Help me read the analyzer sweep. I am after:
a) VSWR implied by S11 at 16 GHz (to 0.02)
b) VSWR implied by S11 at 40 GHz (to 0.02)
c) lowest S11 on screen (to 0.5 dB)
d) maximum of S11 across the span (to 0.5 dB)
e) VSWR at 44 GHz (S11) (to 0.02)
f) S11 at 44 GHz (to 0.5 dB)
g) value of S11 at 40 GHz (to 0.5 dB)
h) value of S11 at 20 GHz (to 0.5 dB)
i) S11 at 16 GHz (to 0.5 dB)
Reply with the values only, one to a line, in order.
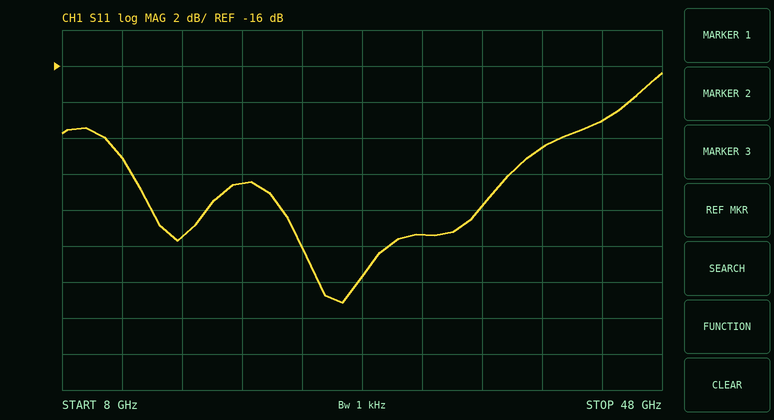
1.12
1.20
-29.0 dB
-16.5 dB
1.26
-19.0 dB
-20.5 dB
-22.5 dB
-25.5 dB
